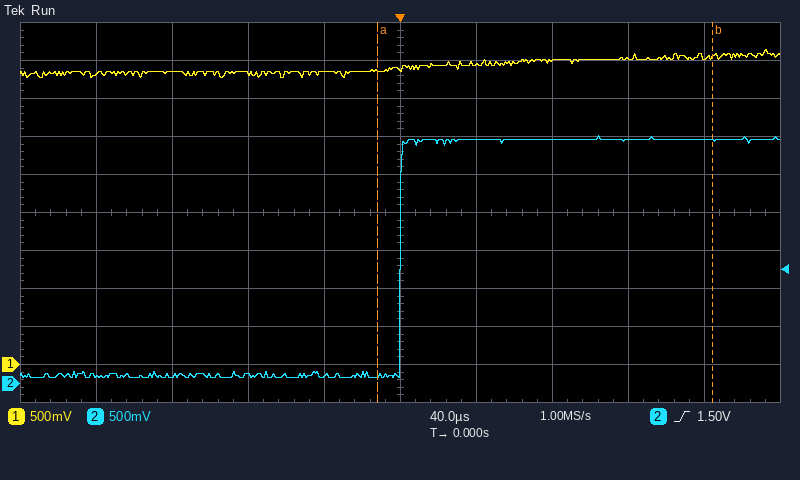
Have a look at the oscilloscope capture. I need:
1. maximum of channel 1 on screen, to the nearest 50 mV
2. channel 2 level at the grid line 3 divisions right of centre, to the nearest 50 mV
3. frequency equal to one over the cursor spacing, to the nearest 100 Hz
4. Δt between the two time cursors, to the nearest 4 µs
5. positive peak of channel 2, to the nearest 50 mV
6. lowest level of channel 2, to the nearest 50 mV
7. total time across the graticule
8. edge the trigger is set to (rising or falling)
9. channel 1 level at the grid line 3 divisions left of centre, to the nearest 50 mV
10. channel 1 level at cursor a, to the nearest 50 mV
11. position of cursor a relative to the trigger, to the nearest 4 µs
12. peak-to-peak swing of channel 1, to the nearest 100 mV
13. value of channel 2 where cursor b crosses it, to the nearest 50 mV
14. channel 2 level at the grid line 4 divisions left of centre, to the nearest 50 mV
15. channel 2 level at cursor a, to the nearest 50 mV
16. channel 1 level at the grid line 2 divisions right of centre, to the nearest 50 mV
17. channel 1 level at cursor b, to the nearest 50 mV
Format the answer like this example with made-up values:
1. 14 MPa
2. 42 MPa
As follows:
1. 4.15 V
2. 3.20 V
3. 5.7 kHz
4. 176 µs
5. 3.25 V
6. 100 mV
7. 400 µs
8. rising
9. 3.85 V
10. 3.85 V
11. -12 µs
12. 400 mV
13. 3.20 V
14. 100 mV
15. 100 mV
16. 4.00 V
17. 4.05 V
